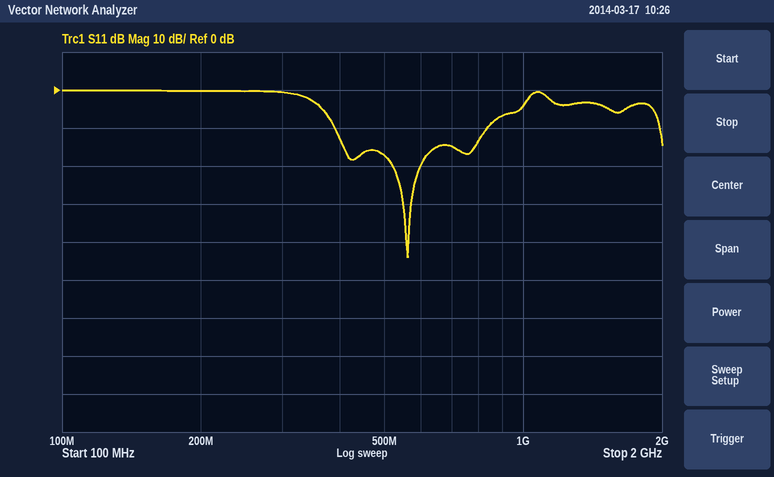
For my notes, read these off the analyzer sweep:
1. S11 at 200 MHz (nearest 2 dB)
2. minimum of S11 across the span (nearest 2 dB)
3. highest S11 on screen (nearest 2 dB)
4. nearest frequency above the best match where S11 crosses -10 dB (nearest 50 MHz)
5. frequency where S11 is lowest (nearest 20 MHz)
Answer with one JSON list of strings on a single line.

["0 dB", "-44 dB", "0 dB", "850 MHz", "560 MHz"]
